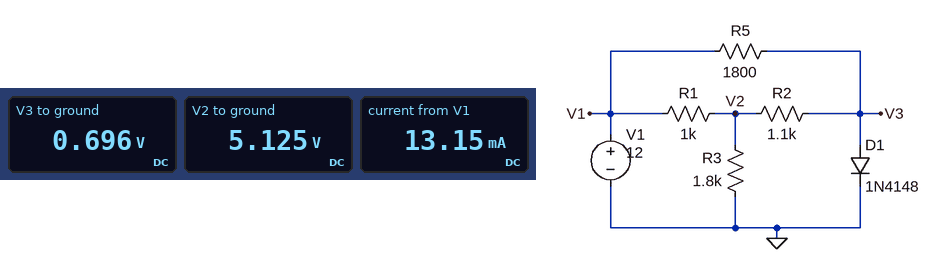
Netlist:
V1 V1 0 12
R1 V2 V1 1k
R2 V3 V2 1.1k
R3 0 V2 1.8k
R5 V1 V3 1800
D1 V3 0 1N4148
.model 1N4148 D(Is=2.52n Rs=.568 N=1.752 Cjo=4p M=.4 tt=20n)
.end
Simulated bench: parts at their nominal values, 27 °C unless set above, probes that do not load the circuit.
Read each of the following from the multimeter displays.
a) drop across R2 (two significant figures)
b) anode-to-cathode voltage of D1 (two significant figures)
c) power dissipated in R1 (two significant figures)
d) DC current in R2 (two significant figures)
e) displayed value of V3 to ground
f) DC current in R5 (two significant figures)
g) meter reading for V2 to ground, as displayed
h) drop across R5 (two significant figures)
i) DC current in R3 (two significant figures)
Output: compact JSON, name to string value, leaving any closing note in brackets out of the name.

{"drop across R2": "4.4 V", "anode-to-cathode voltage of D1": "700 mV", "power dissipated in R1": "47 mW", "DC current in R2": "4.0 mA", "displayed value of V3 to ground": "0.696 V", "DC current in R5": "6.3 mA", "meter reading for V2 to ground, as displayed": "5.125 V", "drop across R5": "11 V", "DC current in R3": "2.8 mA"}
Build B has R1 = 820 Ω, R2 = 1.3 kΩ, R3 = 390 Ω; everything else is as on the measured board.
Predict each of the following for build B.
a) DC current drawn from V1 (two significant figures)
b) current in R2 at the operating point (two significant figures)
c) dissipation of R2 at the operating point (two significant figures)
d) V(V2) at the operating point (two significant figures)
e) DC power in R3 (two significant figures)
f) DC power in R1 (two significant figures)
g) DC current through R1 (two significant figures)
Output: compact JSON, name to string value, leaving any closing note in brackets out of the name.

{"DC current drawn from V1": "17 mA", "current in R2 at the operating point": "2.0 mA", "dissipation of R2 at the operating point": "5.4 mW", "V(V2) at the operating point": "3.3 V", "DC power in R3": "28 mW", "DC power in R1": "92 mW", "DC current through R1": "11 mA"}
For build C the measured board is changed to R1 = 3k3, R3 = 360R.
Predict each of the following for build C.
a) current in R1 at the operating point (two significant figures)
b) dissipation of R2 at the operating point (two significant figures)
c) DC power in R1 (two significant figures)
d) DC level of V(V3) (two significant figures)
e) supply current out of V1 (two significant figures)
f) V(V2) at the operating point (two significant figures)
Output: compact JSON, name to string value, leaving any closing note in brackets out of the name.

{"current in R1 at the operating point": "3.3 mA", "dissipation of R2 at the operating point": "140 µW", "DC power in R1": "36 mW", "DC level of V(V3)": "670 mV", "supply current out of V1": "9.6 mA", "V(V2) at the operating point": "1.1 V"}
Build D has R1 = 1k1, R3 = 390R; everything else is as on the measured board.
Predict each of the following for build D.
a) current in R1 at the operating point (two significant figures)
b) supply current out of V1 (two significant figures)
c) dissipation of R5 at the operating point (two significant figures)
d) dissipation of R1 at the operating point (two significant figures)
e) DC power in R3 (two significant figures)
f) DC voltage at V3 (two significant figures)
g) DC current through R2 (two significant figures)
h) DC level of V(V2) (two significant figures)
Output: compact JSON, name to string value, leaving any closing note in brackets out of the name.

{"current in R1 at the operating point": "8.5 mA", "supply current out of V1": "15 mA", "dissipation of R5 at the operating point": "71 mW", "dissipation of R1 at the operating point": "80 mW", "DC power in R3": "18 mW", "DC voltage at V3": "680 mV", "DC current through R2": "1.8 mA", "DC level of V(V2)": "2.6 V"}
